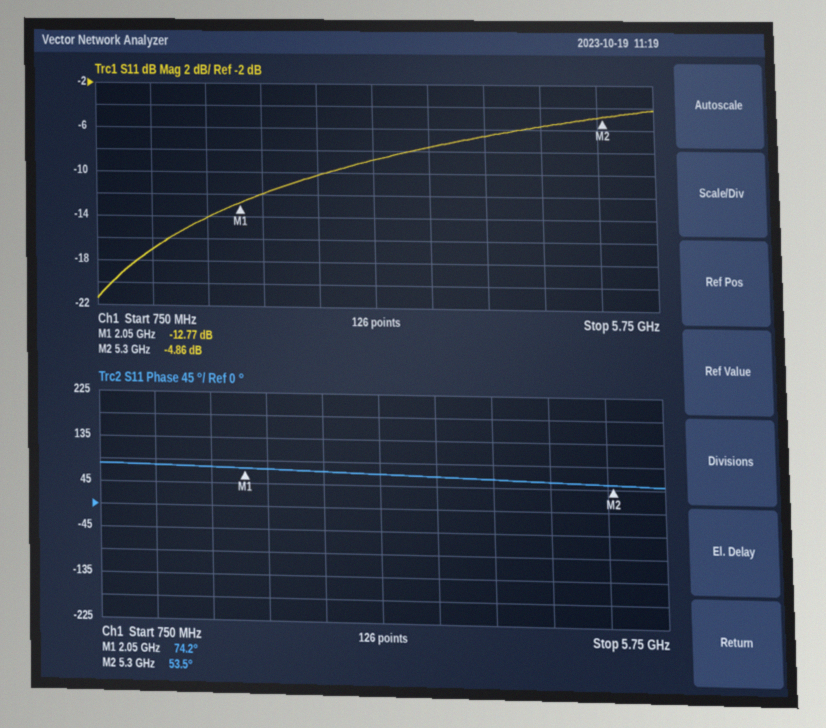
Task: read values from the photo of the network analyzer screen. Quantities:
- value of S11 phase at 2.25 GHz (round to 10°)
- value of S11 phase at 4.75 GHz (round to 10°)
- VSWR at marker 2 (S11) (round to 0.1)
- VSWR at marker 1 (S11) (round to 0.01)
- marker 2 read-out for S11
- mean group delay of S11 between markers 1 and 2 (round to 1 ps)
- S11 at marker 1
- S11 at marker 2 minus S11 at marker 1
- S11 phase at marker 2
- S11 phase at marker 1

70°
60°
3.7
1.60
-4.86 dB
18 ps
-12.77 dB
7.91 dB
53.5°
74.2°
